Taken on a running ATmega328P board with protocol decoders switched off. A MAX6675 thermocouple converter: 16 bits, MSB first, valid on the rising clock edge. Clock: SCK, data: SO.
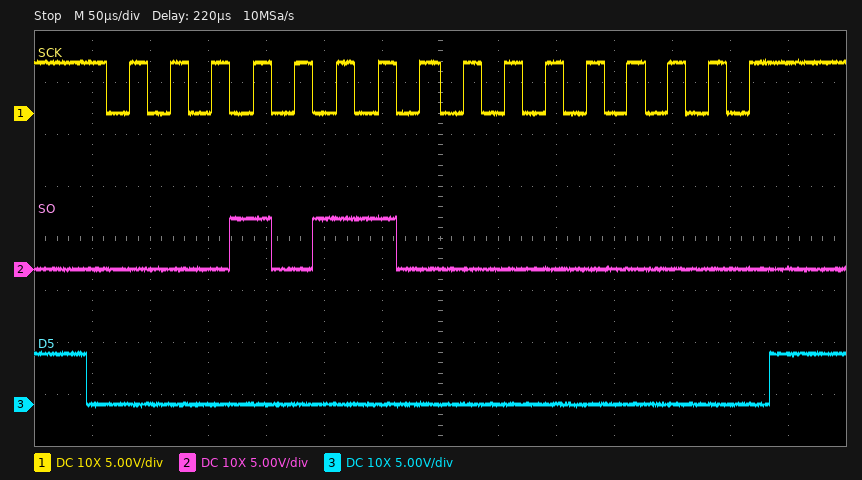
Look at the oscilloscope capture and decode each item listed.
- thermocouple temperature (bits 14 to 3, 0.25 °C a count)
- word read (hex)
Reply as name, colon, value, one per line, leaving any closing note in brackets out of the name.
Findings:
thermocouple temperature: 176.00 °C
word read: 0x1600
